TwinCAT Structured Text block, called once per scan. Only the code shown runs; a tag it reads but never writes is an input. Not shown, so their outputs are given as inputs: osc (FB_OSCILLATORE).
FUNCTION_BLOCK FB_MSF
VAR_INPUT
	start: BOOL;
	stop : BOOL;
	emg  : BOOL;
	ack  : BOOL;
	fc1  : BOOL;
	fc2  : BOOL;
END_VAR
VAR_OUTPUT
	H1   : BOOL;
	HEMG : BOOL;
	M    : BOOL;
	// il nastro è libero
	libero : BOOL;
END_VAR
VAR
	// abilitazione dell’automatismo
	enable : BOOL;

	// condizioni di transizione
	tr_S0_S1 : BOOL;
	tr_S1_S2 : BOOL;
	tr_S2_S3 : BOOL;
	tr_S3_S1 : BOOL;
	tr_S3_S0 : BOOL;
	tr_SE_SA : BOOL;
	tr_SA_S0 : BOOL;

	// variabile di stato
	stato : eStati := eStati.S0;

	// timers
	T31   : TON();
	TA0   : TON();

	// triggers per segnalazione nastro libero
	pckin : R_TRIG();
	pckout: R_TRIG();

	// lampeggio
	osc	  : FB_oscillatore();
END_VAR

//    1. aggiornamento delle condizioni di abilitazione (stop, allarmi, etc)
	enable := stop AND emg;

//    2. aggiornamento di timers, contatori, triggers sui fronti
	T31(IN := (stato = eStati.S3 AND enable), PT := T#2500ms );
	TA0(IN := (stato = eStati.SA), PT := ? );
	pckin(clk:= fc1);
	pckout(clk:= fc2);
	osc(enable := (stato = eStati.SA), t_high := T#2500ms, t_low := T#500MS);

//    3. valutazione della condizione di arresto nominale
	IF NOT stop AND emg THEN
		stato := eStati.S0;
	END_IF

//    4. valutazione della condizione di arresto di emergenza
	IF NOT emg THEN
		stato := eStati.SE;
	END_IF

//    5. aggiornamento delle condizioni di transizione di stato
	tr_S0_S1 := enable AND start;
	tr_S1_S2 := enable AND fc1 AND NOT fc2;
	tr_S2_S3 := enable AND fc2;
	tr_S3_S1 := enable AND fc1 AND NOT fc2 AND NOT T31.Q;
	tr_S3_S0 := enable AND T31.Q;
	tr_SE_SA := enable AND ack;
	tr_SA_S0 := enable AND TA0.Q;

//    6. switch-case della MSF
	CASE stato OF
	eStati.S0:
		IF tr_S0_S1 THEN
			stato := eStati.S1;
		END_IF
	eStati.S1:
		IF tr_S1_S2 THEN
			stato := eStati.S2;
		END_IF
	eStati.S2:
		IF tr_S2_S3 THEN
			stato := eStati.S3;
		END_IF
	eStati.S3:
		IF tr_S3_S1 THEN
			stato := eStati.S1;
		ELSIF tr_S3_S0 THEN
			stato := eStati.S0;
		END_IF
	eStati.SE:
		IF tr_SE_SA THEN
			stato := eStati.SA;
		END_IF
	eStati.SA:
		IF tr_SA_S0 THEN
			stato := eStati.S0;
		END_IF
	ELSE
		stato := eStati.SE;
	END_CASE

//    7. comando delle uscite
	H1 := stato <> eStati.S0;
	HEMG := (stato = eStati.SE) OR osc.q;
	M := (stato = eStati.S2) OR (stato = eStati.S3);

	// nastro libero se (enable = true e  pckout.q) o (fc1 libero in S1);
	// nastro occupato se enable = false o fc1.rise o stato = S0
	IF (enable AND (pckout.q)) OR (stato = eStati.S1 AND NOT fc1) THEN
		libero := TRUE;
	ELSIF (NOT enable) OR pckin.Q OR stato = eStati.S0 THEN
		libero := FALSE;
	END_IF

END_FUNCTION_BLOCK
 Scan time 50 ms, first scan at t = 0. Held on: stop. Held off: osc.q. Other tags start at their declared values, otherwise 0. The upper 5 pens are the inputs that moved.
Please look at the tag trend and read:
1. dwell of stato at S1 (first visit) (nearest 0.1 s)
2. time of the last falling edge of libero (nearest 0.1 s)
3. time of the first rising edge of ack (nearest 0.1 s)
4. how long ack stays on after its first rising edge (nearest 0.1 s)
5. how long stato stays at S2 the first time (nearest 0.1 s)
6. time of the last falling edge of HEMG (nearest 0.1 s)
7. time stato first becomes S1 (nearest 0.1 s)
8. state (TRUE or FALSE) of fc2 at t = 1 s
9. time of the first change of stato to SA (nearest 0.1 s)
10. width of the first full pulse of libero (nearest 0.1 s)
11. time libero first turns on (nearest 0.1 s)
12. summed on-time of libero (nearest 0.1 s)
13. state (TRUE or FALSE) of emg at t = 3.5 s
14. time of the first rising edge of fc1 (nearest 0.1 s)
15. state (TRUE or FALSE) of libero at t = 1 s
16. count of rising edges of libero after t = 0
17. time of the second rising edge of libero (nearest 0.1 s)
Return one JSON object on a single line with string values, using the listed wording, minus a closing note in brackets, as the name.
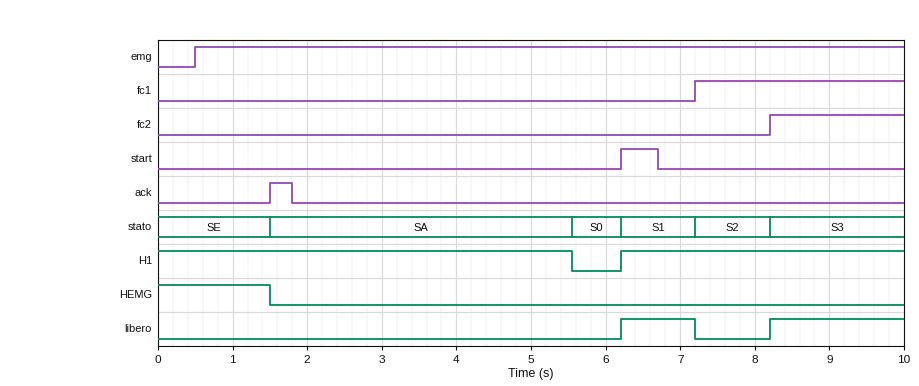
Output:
{"dwell of stato at S1 (first visit)": "1.0 s", "time of the last falling edge of libero": "7.2 s", "time of the first rising edge of ack": "1.5 s", "how long ack stays on after its first rising edge": "0.3 s", "how long stato stays at S2 the first time": "1.0 s", "time of the last falling edge of HEMG": "1.5 s", "time stato first becomes S1": "6.2 s", "state (TRUE or FALSE) of fc2 at t = 1 s": "FALSE", "time of the first change of stato to SA": "1.5 s", "width of the first full pulse of libero": "1.0 s", "time libero first turns on": "6.2 s", "summed on-time of libero": "2.8 s", "state (TRUE or FALSE) of emg at t = 3.5 s": "TRUE", "time of the first rising edge of fc1": "7.2 s", "state (TRUE or FALSE) of libero at t = 1 s": "FALSE", "count of rising edges of libero after t = 0": "2", "time of the second rising edge of libero": "8.2 s"}
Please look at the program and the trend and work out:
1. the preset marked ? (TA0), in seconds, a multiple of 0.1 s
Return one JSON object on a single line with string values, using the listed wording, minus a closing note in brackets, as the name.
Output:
{"the preset marked ? (TA0), in seconds, a multiple of 0.1 s": "4.0 s"}
